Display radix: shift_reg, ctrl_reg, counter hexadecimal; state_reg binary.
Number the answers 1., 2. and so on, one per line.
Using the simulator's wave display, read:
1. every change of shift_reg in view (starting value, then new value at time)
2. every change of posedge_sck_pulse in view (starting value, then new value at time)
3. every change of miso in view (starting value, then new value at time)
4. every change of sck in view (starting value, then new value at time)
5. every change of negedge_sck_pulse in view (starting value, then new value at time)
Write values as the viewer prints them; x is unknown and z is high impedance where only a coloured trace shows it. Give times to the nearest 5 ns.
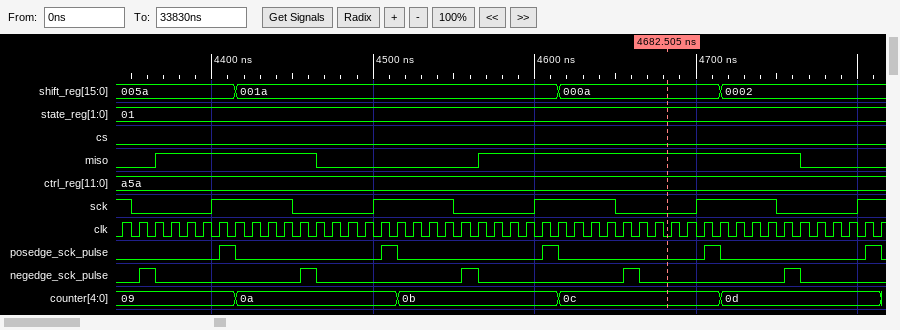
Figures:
1. 005a, 001a at 4415 ns, 000a at 4615 ns, 0002 at 4715 ns
2. 0, 1 at 4405 ns, 0 at 4415 ns, 1 at 4505 ns, 0 at 4515 ns, 1 at 4605 ns, 0 at 4615 ns, 1 at 4705 ns, 0 at 4715 ns, 1 at 4805 ns, 0 at 4815 ns
3. 0, 1 at 4365 ns, 0 at 4465 ns, 1 at 4565 ns, 0 at 4765 ns
4. 1, 0 at 4350 ns, 1 at 4400 ns, 0 at 4450 ns, 1 at 4500 ns, 0 at 4550 ns, 1 at 4600 ns, 0 at 4650 ns, 1 at 4700 ns, 0 at 4750 ns, 1 at 4800 ns
5. 0, 1 at 4355 ns, 0 at 4365 ns, 1 at 4455 ns, 0 at 4465 ns, 1 at 4555 ns, 0 at 4565 ns, 1 at 4655 ns, 0 at 4665 ns, 1 at 4755 ns, 0 at 4765 ns
